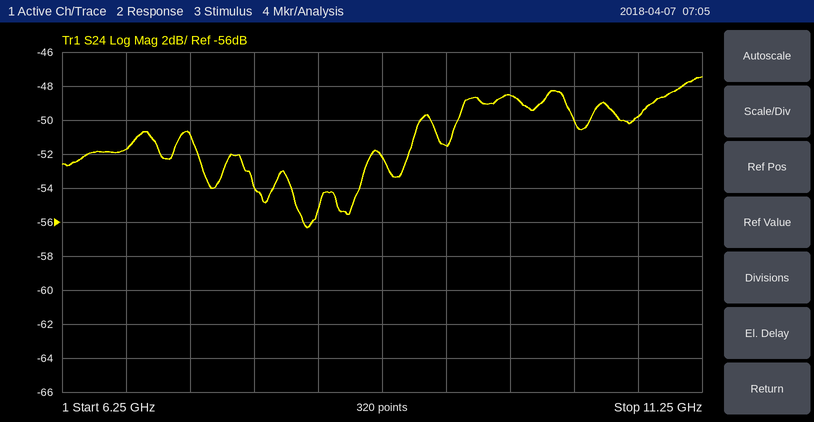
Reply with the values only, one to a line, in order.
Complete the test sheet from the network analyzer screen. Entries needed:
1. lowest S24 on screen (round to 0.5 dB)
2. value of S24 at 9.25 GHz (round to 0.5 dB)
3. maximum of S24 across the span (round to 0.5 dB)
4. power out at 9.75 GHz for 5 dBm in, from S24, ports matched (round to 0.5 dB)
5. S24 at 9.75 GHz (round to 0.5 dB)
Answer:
-56.5 dB
-51.5 dB
-47.5 dB
-43.5 dBm
-48.5 dB
